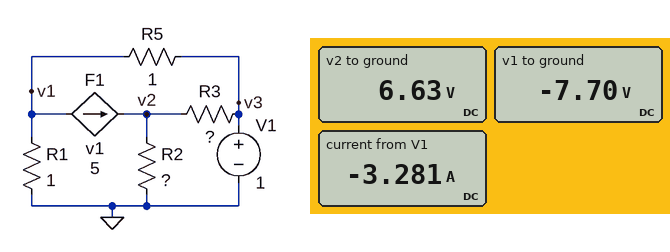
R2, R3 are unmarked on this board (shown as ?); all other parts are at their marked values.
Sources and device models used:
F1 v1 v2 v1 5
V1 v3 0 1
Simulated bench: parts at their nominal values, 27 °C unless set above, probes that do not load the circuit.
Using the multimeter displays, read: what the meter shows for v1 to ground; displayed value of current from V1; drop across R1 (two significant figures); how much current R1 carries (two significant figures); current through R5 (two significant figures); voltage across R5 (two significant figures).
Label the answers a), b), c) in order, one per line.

a) -7.70 V
b) -3.281 A
c) 7.7 V
d) 7.7 A
e) 8.7 A
f) 8.7 V
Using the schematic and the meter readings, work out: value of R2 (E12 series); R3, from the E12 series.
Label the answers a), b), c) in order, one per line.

a) 1.5 Ω
b) 0.47 Ω
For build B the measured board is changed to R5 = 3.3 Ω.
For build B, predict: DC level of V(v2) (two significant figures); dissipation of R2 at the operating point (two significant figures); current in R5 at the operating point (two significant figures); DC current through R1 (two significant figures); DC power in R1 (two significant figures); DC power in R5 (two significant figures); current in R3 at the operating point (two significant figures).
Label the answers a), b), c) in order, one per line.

a) 1.6 V
b) 1.6 W
c) 760 mA
d) 1.5 A
e) 2.2 W
f) 1.9 W
g) 1.2 A
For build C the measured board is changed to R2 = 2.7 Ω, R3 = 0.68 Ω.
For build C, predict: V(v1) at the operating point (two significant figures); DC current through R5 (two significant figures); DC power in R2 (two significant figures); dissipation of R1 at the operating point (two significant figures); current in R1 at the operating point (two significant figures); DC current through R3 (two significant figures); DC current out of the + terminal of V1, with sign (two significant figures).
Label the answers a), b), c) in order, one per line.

a) -3.5 V
b) 4.5 A
c) 9.9 W
d) 12 W
e) 3.5 A
f) 6.1 A
g) -1.6 A
